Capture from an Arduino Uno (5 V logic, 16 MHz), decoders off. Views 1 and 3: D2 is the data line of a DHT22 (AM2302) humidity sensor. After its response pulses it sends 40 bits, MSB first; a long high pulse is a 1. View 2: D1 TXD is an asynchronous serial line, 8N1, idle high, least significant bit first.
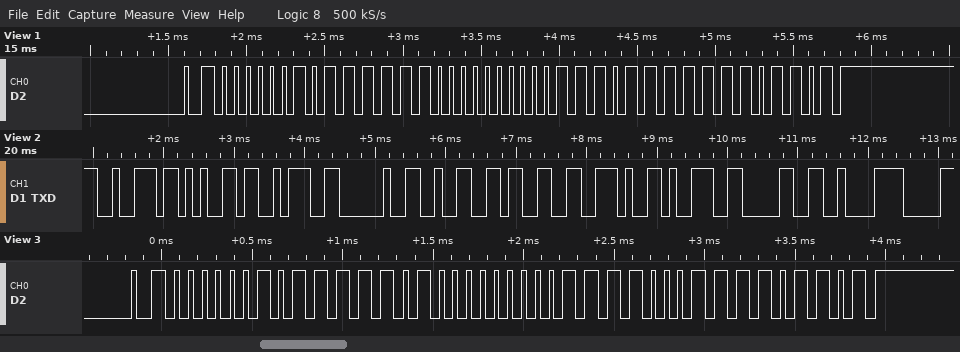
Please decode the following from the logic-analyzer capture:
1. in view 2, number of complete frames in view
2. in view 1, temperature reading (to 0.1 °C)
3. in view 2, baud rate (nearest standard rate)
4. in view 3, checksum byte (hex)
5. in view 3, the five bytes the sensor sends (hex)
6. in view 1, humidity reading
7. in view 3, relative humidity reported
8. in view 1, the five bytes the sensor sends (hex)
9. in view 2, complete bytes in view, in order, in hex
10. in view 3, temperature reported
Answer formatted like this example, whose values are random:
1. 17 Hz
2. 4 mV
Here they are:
1. 10
2. 23.9 °C
3. 9600 baud
4. 0xED
5. 02 FA 00 F1 ED
6. 76.4 %
7. 76.2 %
8. 02 FC 00 EF ED
9. 72 65 3A 20 32 33 2E 39 30 C2
10. 24.1 °C
